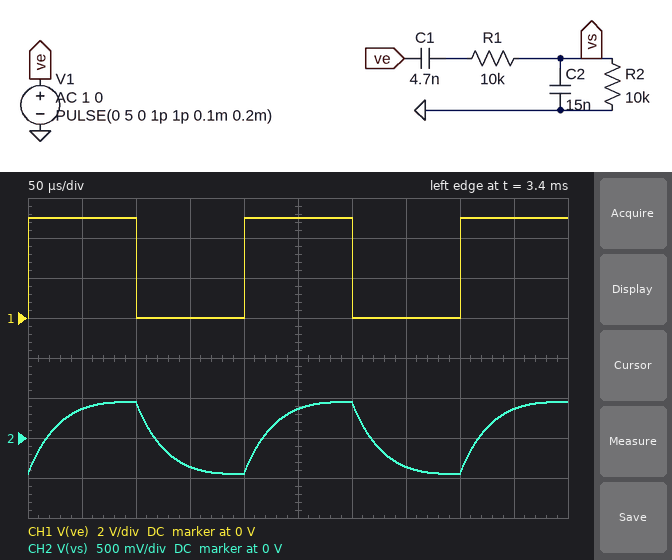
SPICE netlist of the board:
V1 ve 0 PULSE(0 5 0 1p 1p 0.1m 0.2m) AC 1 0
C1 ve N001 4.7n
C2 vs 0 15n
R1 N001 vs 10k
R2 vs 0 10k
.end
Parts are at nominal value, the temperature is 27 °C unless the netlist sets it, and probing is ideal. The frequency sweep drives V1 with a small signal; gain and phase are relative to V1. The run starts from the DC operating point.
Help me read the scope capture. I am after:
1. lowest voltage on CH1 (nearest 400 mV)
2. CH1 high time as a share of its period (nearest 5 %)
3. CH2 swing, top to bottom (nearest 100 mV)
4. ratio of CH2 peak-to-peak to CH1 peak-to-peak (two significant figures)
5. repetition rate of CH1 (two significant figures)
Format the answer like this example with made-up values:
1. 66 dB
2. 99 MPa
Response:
1. 0 V
2. 50 %
3. 900 mV
4. 0.18
5. 5.0 kHz
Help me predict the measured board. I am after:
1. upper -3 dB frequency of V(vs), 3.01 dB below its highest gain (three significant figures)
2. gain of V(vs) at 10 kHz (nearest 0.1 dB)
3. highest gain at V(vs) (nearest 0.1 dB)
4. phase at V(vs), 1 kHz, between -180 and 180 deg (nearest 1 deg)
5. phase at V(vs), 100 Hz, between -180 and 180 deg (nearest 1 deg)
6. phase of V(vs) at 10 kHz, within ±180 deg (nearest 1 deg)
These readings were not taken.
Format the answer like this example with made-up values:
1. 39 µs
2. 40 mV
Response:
1. 6.10 kHz
2. -20.4 dB
3. -14.3 dB
4. 25 deg
5. 81 deg
6. -60 deg
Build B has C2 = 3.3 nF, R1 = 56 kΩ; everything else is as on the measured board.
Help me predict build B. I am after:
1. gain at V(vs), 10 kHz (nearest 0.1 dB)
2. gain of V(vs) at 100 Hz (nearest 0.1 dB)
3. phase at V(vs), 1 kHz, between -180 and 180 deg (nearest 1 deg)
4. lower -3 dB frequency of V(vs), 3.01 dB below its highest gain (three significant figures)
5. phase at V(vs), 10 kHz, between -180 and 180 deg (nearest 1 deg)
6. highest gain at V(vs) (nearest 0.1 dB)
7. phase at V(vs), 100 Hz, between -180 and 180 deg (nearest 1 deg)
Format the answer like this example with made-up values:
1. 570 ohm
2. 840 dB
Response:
1. -22.6 dB
2. -30.8 dB
3. 17 deg
4. 434 Hz
5. -57 deg
6. -17.3 dB
7. 78 deg
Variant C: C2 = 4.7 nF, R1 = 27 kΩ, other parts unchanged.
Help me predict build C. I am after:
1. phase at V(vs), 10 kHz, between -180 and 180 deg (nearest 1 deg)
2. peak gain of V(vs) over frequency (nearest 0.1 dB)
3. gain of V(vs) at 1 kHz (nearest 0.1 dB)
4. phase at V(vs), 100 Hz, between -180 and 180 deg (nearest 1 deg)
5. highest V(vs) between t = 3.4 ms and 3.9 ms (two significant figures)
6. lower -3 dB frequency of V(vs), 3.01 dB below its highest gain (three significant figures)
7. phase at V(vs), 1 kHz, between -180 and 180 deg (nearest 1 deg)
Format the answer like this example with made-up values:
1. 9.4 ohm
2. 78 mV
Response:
1. -58 deg
2. -13.4 dB
3. -14.6 dB
4. 82 deg
5. 500 mV
6. 649 Hz
7. 29 deg
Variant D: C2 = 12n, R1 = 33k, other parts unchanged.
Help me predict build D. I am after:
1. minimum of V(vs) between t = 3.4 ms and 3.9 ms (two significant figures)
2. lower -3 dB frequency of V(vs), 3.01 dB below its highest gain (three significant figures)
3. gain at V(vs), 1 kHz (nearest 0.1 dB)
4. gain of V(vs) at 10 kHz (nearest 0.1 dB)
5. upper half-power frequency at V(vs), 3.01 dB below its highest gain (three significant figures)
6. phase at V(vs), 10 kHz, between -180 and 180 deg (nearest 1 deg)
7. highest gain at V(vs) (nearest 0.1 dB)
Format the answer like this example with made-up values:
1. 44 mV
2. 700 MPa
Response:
1. -260 mV
2. 428 Hz
3. -16.8 dB
4. -28.1 dB
5. 3.18 kHz
6. -74 deg
7. -16.7 dB
